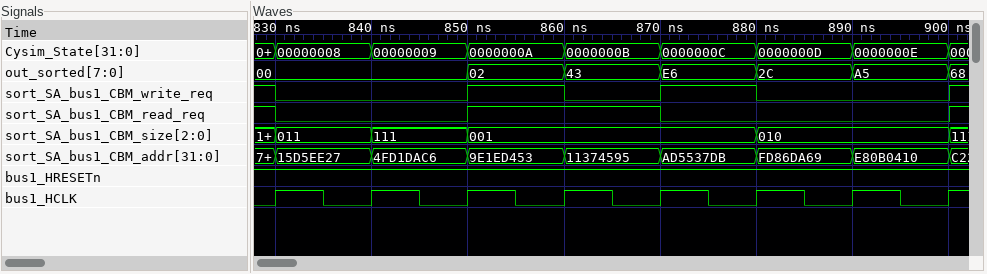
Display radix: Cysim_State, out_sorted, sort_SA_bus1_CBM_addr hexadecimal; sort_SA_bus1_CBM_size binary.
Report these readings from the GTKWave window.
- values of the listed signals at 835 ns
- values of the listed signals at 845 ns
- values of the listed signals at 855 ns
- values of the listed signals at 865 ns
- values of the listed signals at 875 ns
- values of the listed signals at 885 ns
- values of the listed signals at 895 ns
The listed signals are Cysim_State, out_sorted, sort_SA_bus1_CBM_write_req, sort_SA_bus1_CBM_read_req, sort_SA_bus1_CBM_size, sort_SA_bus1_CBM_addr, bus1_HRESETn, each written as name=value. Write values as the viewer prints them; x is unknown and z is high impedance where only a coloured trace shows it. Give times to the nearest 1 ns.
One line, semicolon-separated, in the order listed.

Cysim_State=00000008, out_sorted=00, sort_SA_bus1_CBM_write_req=0, sort_SA_bus1_CBM_read_req=0, sort_SA_bus1_CBM_size=011, sort_SA_bus1_CBM_addr=15D5EE27, bus1_HRESETn=1; Cysim_State=00000009, out_sorted=00, sort_SA_bus1_CBM_write_req=0, sort_SA_bus1_CBM_read_req=0, sort_SA_bus1_CBM_size=111, sort_SA_bus1_CBM_addr=4FD1DAC6, bus1_HRESETn=1; Cysim_State=0000000A, out_sorted=02, sort_SA_bus1_CBM_write_req=1, sort_SA_bus1_CBM_read_req=1, sort_SA_bus1_CBM_size=001, sort_SA_bus1_CBM_addr=9E1ED453, bus1_HRESETn=1; Cysim_State=0000000B, out_sorted=43, sort_SA_bus1_CBM_write_req=0, sort_SA_bus1_CBM_read_req=1, sort_SA_bus1_CBM_size=001, sort_SA_bus1_CBM_addr=11374595, bus1_HRESETn=1; Cysim_State=0000000C, out_sorted=E6, sort_SA_bus1_CBM_write_req=1, sort_SA_bus1_CBM_read_req=0, sort_SA_bus1_CBM_size=001, sort_SA_bus1_CBM_addr=AD5537DB, bus1_HRESETn=1; Cysim_State=0000000D, out_sorted=2C, sort_SA_bus1_CBM_write_req=0, sort_SA_bus1_CBM_read_req=0, sort_SA_bus1_CBM_size=010, sort_SA_bus1_CBM_addr=FD86DA69, bus1_HRESETn=1; Cysim_State=0000000E, out_sorted=A5, sort_SA_bus1_CBM_write_req=0, sort_SA_bus1_CBM_read_req=0, sort_SA_bus1_CBM_size=010, sort_SA_bus1_CBM_addr=E80B0410, bus1_HRESETn=1
